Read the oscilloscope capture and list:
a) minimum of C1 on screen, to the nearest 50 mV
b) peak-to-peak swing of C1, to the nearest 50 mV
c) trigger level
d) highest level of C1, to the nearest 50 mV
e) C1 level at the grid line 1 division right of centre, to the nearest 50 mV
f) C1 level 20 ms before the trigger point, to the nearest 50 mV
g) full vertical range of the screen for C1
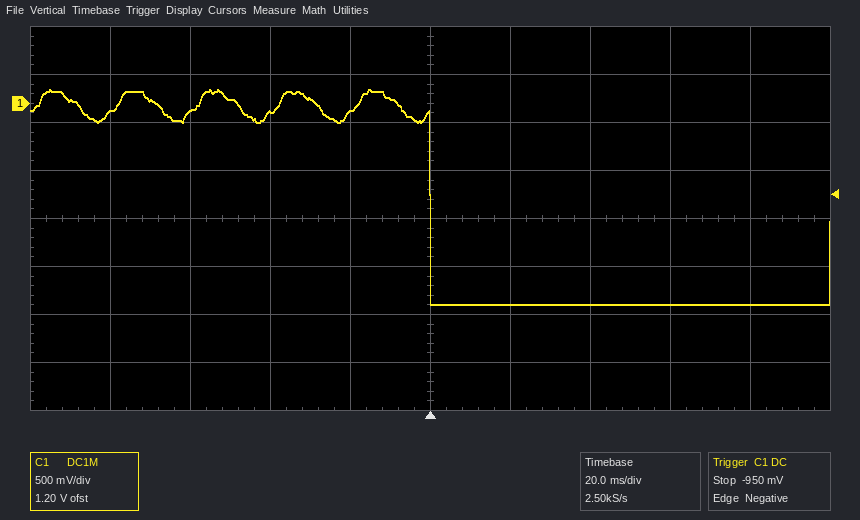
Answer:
-2.10 V
2.25 V
-950 mV
150 mV
-2.10 V
-100 mV
4 V
